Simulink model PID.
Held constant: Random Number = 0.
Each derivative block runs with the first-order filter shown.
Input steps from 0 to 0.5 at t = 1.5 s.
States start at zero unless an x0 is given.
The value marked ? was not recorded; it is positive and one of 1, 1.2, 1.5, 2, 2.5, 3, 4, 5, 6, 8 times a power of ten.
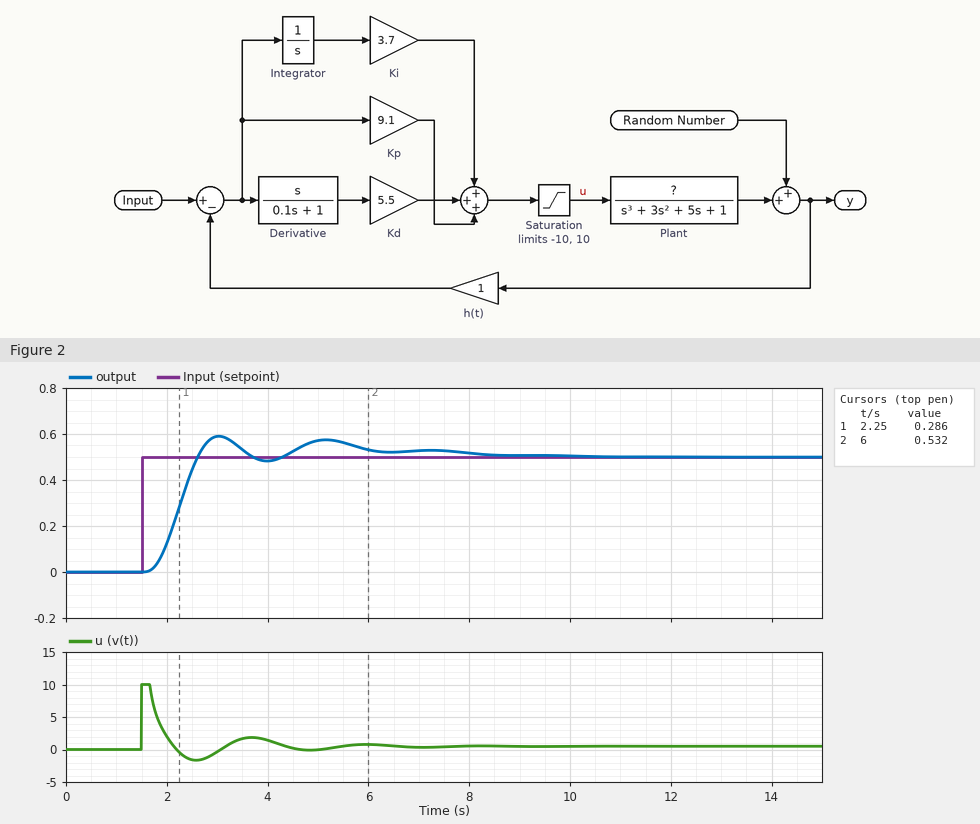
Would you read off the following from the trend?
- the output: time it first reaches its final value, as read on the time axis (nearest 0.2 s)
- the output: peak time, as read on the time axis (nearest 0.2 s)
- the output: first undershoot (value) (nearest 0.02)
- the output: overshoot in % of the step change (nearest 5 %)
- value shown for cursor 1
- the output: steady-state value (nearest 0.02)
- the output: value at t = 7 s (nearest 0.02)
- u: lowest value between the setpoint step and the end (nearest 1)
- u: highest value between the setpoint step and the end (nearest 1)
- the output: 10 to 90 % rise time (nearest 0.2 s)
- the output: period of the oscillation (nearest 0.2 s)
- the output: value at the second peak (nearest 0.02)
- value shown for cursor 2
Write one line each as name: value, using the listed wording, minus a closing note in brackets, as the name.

the output: time it first reaches its final value, as read on the time axis: 2.6 s
the output: peak time, as read on the time axis: 3.0 s
the output: first undershoot (value): 0.48
the output: overshoot in % of the step change: 20 %
value shown for cursor 1: 0.286
the output: steady-state value: 0.50
the output: value at t = 7 s: 0.52
u: lowest value between the setpoint step and the end: -2
u: highest value between the setpoint step and the end: 10
the output: 10 to 90 % rise time: 0.6 s
the output: period of the oscillation: 2.2 s
the output: value at the second peak: 0.58
value shown for cursor 2: 0.532
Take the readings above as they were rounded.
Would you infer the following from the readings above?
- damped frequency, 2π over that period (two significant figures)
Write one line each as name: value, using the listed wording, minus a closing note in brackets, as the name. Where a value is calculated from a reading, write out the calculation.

damped frequency, 2π over that period: 2π / 2.2 = 2.9 rad/s
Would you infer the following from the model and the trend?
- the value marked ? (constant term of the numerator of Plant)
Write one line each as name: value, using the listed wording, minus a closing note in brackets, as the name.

the value marked ?: 1
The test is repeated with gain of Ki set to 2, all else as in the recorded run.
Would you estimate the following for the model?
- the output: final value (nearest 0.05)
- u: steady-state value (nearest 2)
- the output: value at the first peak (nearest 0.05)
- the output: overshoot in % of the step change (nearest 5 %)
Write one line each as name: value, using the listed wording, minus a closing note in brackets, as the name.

the output: final value: 0.50
u: steady-state value: 0
the output: value at the first peak: 0.55
the output: overshoot in % of the step change: 10 %
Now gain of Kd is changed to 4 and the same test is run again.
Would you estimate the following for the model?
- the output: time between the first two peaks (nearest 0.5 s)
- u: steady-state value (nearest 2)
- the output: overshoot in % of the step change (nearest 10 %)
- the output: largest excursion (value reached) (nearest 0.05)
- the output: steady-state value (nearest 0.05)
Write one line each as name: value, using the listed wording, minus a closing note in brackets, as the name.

the output: time between the first two peaks: 2.5 s
u: steady-state value: 0
the output: overshoot in % of the step change: 30 %
the output: largest excursion (value reached): 0.65
the output: steady-state value: 0.50
